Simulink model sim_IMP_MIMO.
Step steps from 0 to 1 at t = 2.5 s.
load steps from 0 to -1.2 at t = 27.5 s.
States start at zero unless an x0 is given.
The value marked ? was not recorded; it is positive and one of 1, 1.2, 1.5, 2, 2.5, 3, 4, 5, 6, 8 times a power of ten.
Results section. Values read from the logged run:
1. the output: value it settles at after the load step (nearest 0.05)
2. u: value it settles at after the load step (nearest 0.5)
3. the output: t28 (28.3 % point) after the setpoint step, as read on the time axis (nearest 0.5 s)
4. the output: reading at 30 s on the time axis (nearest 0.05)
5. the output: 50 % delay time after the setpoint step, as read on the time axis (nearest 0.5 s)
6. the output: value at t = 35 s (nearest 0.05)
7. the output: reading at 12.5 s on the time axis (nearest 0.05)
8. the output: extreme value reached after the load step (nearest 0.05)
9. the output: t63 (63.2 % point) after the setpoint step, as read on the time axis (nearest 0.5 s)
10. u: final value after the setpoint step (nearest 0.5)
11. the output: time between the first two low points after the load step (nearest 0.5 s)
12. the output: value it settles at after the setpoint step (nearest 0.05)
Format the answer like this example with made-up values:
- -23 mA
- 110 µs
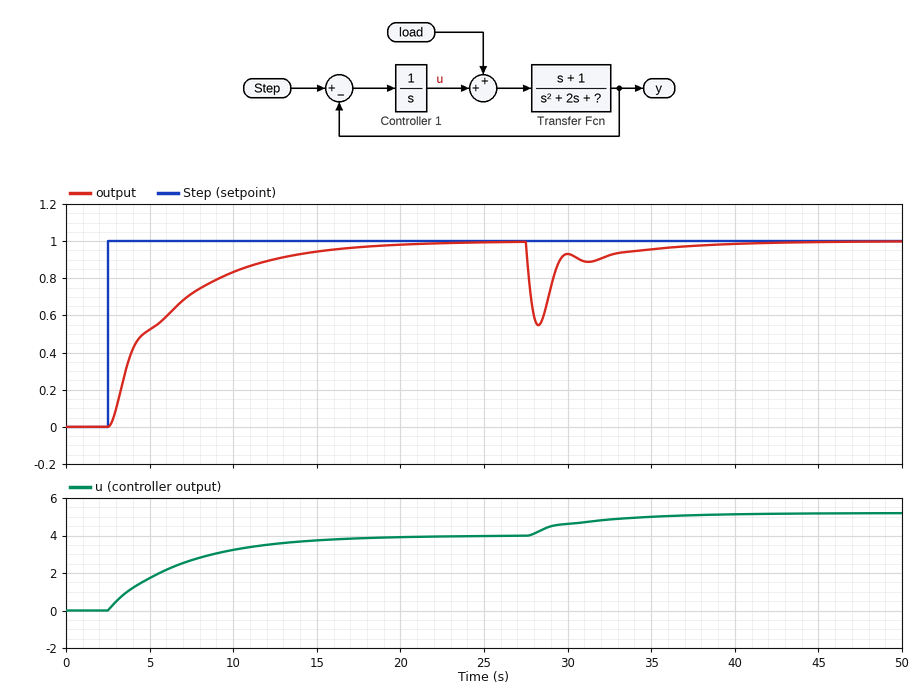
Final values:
- 1.00
- 5.0
- 3.5 s
- 0.95
- 4.5 s
- 0.95
- 0.90
- 0.55
- 6.5 s
- 4.0
- 3.0 s
- 1.00
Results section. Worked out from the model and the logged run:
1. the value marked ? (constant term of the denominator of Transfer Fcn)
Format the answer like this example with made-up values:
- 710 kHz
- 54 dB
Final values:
- 4
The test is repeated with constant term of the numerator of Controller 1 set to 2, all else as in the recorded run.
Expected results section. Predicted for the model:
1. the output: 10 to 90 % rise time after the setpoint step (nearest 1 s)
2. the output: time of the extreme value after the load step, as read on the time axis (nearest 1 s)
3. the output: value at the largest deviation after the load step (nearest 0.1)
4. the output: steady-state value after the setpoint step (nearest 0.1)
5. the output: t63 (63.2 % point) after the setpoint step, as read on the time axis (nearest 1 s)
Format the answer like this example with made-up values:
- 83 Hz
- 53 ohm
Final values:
- 5 s
- 28 s
- 0.6
- 1.0
- 4 s
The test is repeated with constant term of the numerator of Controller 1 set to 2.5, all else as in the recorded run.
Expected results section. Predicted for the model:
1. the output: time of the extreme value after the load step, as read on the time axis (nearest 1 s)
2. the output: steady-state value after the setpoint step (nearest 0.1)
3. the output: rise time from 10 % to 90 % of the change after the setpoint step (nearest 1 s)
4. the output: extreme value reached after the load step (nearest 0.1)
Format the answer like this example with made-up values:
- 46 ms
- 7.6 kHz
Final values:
- 28 s
- 1.0
- 4 s
- 0.6
